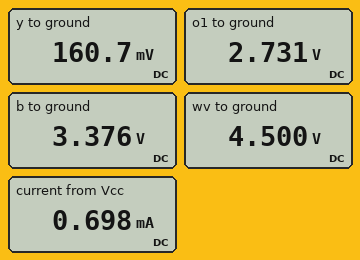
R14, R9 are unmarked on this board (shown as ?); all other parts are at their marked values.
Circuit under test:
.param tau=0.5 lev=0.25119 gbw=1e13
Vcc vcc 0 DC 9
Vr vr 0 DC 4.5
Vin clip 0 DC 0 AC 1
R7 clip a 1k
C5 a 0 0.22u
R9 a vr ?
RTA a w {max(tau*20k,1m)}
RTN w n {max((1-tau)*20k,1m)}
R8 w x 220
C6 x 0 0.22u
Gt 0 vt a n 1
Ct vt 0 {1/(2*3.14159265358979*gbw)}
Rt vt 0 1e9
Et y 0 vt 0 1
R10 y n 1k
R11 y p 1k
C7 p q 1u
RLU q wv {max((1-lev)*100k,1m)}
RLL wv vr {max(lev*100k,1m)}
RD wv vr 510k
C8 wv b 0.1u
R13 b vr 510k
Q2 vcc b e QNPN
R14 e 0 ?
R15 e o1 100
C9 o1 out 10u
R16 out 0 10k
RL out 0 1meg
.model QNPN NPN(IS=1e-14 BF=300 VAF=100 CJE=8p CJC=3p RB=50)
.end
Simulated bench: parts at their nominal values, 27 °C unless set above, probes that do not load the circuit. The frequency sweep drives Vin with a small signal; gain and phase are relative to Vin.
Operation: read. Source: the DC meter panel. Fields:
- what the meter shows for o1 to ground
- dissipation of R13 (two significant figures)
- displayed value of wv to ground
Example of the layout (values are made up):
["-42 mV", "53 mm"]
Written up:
["2.731 V", "2.5 µW", "4.500 V"]
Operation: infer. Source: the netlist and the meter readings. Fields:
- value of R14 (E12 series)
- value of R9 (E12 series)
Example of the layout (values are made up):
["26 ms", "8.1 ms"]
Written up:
["3.9 kΩ", "27 kΩ"]
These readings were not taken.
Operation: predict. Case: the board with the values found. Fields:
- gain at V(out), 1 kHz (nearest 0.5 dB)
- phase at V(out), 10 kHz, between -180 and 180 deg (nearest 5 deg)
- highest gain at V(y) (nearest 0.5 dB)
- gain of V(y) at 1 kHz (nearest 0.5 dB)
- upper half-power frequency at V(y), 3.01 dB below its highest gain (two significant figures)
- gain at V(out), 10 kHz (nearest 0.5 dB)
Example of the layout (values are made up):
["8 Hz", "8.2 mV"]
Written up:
["-17.5 dB", "-85 deg", "-0.5 dB", "-4.5 dB", "810 Hz", "-35.0 dB"]
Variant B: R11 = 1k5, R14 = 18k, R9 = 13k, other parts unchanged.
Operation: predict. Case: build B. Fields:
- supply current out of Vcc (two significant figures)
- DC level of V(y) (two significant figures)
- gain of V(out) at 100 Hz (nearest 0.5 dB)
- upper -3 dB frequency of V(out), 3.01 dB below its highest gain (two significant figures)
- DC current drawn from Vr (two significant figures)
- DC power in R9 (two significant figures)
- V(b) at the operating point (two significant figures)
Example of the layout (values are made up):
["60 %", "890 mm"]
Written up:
["200 µA", "320 mV", "-14.0 dB", "860 Hz", "320 µA", "1.3 mW", "4.2 V"]
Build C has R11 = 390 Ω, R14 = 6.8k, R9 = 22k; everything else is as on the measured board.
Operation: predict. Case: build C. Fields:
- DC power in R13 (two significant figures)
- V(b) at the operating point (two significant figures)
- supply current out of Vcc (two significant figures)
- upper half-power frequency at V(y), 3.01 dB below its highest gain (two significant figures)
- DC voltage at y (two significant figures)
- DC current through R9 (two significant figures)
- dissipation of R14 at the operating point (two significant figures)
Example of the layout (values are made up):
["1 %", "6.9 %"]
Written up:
["1.1 µW", "3.8 V", "460 µA", "820 Hz", "200 mV", "200 µA", "1.4 mW"]
